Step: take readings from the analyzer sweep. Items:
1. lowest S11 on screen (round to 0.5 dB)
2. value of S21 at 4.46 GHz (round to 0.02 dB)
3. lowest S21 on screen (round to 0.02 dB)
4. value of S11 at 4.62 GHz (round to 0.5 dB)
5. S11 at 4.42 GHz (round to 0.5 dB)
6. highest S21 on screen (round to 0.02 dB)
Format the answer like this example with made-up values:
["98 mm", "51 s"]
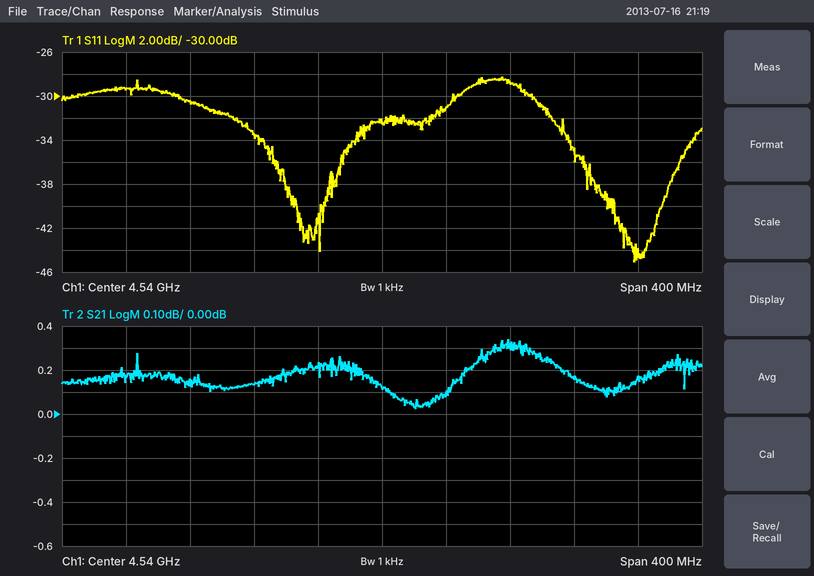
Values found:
["-45.0 dB", "0.14 dB", "0.02 dB", "-29.0 dB", "-30.5 dB", "0.34 dB"]
